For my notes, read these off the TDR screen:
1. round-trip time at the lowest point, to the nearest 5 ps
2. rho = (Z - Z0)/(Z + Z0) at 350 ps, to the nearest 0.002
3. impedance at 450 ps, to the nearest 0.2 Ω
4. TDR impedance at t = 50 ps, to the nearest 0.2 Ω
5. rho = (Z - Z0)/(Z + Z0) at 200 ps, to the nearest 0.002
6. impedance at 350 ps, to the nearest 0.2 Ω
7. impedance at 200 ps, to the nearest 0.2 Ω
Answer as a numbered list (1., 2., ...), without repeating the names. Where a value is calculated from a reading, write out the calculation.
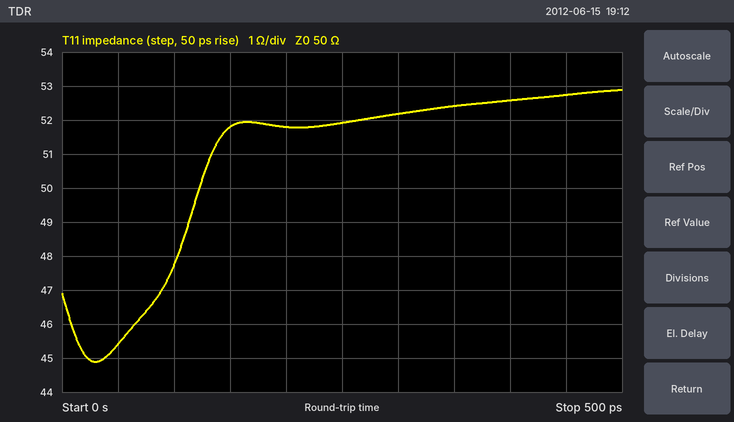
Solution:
1. 30 ps
2. (52.4 − 50)/(52.4 + 50) ≈ +0.0234, so +0.024 to the nearest 0.002
3. 52.8 Ω
4. 45.4 Ω
5. (51.8 − 50)/(51.8 + 50) ≈ +0.018
6. 52.4 Ω
7. 51.8 Ω
